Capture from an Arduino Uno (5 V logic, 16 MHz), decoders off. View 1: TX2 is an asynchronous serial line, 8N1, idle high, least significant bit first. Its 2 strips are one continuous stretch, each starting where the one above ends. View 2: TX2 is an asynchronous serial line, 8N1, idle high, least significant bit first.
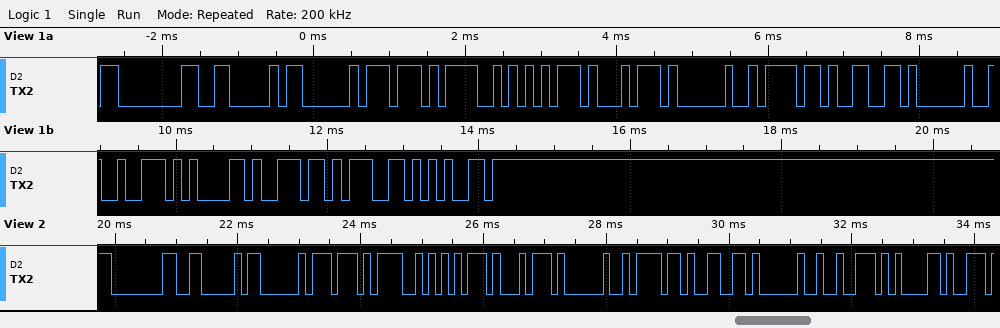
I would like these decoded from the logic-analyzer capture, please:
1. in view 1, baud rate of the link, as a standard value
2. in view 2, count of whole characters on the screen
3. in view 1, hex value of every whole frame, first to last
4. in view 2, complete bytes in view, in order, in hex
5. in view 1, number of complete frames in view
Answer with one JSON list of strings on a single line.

["9600 baud", "13", "80 06 03 77 4F 75 74 20 6F 66 20 72 61 6E 67 65", "80 06 03 77 4F 75 74 20 6F 66 20 72 61", "16"]
